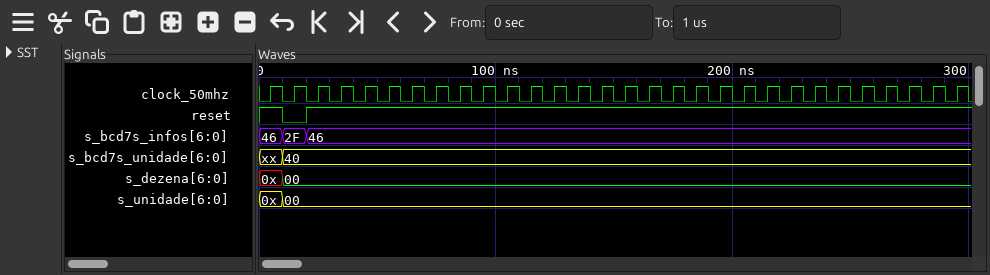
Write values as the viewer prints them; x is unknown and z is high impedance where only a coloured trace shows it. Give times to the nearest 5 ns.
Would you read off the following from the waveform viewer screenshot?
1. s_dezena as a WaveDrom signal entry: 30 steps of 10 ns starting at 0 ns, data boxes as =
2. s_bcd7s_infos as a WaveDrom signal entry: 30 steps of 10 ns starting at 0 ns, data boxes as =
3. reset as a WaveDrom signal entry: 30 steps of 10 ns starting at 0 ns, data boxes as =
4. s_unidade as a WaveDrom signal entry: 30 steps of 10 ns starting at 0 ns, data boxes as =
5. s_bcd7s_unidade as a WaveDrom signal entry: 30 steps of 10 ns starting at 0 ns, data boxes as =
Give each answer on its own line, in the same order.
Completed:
{name: 's_dezena', wave: '==............................', data: '0x 00'}
{name: 's_bcd7s_infos', wave: '===...........................', data: '46 2F 46'}
{name: 'reset', wave: '101...........................'}
{name: 's_unidade', wave: '==............................', data: '0x 00'}
{name: 's_bcd7s_unidade', wave: '==............................', data: 'xx 40'}
